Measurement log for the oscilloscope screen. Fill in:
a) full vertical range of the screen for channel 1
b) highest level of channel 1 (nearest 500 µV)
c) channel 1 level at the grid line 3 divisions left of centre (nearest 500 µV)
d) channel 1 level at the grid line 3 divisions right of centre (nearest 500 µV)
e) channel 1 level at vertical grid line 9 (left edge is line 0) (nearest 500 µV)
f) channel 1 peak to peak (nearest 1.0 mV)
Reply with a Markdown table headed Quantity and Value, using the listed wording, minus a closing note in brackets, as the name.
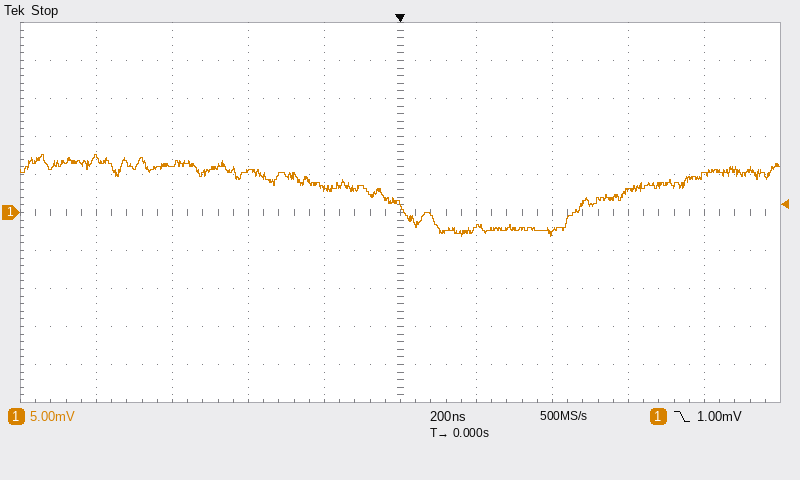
| Quantity | Value |
|---|---|
| full vertical range of the screen for channel 1 | 50 mV |
| highest level of channel 1 | 7.5 mV |
| channel 1 level at the grid line 3 divisions left of centre | 6.5 mV |
| channel 1 level at the grid line 3 divisions right of centre | 3.0 mV |
| channel 1 level at vertical grid line 9 (left edge is line 0) | 5.0 mV |
| channel 1 peak to peak | 11.0 mV |
